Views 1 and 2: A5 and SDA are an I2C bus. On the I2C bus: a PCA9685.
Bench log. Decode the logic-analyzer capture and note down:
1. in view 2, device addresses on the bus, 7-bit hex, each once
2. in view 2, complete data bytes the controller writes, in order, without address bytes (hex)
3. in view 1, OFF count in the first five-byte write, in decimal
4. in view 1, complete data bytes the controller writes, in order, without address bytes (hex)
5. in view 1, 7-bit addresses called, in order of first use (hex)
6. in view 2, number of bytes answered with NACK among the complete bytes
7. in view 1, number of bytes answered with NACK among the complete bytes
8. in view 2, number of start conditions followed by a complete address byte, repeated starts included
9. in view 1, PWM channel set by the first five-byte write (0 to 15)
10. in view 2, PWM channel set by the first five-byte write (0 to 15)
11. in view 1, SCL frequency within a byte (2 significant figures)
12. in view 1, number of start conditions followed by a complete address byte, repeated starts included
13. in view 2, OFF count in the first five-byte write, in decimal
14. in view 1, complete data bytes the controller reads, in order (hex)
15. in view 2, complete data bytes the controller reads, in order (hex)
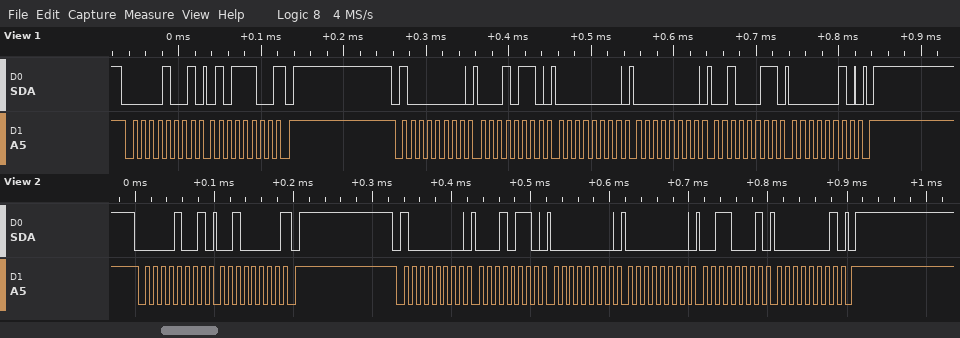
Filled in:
0x04 0x40
16 00 00 31 01
547
16 00 00 23 02
0x04 0x40
1
1
2
4
4
100 kHz
2
305
5C
20
